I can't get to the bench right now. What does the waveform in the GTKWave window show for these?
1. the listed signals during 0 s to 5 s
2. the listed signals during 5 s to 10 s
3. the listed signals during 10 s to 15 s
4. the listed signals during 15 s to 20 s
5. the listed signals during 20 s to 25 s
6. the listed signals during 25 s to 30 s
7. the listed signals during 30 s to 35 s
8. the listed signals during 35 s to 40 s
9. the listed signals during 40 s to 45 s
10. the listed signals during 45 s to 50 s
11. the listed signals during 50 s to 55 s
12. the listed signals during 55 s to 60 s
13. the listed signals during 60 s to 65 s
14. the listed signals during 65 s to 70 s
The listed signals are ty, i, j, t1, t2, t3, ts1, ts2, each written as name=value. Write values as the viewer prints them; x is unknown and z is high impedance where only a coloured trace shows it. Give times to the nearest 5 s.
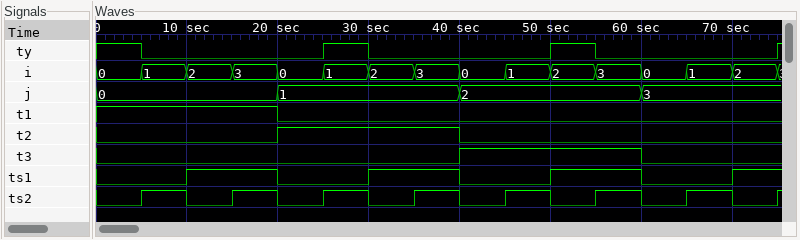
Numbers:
ty=1, i=0, j=0, t1=1, t2=0, t3=0, ts1=0, ts2=0
ty=0, i=1, j=0, t1=1, t2=0, t3=0, ts1=0, ts2=1
ty=0, i=2, j=0, t1=1, t2=0, t3=0, ts1=1, ts2=0
ty=0, i=3, j=0, t1=1, t2=0, t3=0, ts1=1, ts2=1
ty=0, i=0, j=1, t1=0, t2=1, t3=0, ts1=0, ts2=0
ty=1, i=1, j=1, t1=0, t2=1, t3=0, ts1=0, ts2=1
ty=0, i=2, j=1, t1=0, t2=1, t3=0, ts1=1, ts2=0
ty=0, i=3, j=1, t1=0, t2=1, t3=0, ts1=1, ts2=1
ty=0, i=0, j=2, t1=0, t2=0, t3=1, ts1=0, ts2=0
ty=0, i=1, j=2, t1=0, t2=0, t3=1, ts1=0, ts2=1
ty=1, i=2, j=2, t1=0, t2=0, t3=1, ts1=1, ts2=0
ty=0, i=3, j=2, t1=0, t2=0, t3=1, ts1=1, ts2=1
ty=0, i=0, j=3, t1=0, t2=0, t3=0, ts1=0, ts2=0
ty=0, i=1, j=3, t1=0, t2=0, t3=0, ts1=0, ts2=1
